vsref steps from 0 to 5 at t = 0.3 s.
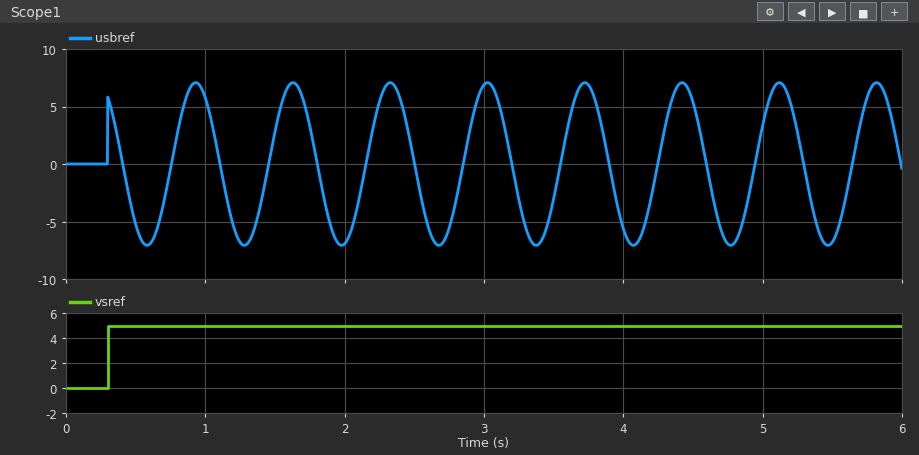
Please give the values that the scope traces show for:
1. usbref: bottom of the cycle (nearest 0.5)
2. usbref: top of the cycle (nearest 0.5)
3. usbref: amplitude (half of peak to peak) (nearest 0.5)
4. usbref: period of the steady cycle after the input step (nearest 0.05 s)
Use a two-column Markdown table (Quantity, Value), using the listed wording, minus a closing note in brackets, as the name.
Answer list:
| Quantity | Value |
|---|---|
| usbref: bottom of the cycle | -7.0 |
| usbref: top of the cycle | 7.0 |
| usbref: amplitude (half of peak to peak) | 7.0 |
| usbref: period of the steady cycle after the input step | 0.70 s |
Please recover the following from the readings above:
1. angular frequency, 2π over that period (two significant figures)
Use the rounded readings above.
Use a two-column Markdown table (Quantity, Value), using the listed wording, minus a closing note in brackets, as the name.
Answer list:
| Quantity | Value |
|---|---|
| angular frequency, 2π over that period | 9.0 rad/s |
